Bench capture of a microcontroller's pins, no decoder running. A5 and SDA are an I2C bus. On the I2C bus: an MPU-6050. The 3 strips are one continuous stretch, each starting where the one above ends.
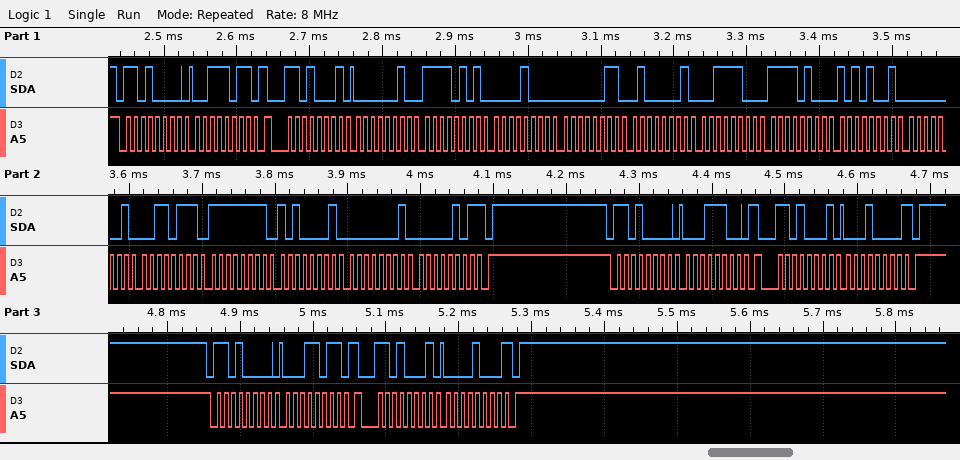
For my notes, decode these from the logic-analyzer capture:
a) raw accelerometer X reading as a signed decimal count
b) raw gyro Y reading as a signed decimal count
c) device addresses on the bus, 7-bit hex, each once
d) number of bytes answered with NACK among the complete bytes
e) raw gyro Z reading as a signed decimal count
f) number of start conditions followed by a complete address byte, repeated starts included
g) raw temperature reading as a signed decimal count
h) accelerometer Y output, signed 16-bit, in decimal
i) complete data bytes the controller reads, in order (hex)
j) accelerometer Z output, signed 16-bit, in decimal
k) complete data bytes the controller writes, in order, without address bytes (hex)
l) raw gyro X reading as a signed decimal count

757
-95
0x68
3
261
6
-2903
2051
02 F5 08 03 41 3C F4 A9 01 37 FF A1 01 05 10 08
16700
3B 1C 1B
311
